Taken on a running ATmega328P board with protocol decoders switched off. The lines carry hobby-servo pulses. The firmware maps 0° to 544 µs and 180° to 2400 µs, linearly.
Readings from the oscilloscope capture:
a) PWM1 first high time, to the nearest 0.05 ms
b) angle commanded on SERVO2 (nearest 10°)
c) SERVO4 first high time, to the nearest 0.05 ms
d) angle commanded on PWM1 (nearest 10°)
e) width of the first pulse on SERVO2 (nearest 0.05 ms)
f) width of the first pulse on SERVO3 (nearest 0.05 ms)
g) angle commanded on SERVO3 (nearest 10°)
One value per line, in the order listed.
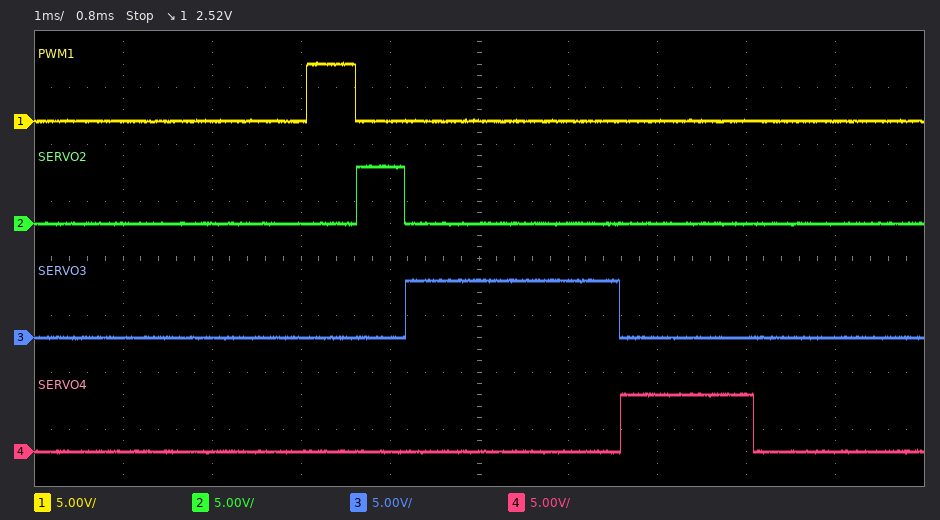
0.55 ms
0°
1.50 ms
0°
0.55 ms
2.40 ms
180°
